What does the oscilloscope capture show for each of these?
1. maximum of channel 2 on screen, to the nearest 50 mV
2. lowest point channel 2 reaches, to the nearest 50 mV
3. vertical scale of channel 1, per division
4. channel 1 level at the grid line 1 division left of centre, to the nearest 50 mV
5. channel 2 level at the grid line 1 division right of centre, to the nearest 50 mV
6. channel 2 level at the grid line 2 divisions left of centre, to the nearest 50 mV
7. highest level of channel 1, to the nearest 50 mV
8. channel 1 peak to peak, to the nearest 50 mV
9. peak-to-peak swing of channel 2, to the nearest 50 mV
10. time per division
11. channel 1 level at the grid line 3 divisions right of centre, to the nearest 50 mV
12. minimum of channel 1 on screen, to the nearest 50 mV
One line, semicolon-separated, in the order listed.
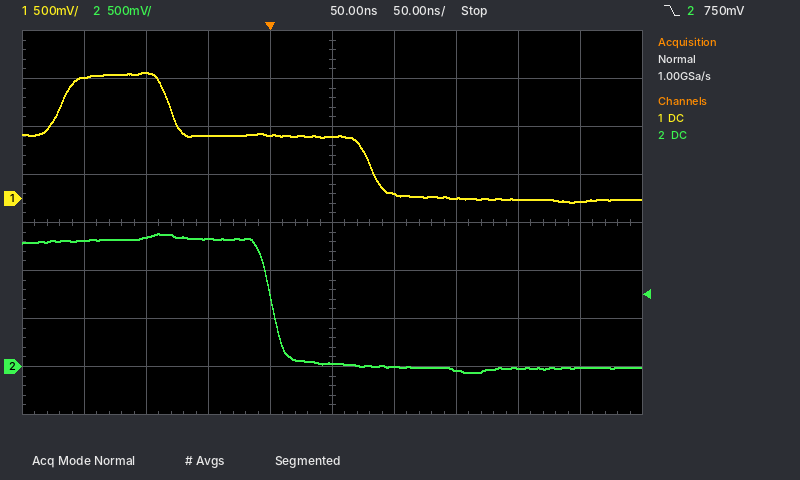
1.40 V; -50 mV; 500 mV; 650 mV; 0 mV; 1.35 V; 1.30 V; 1.35 V; 1.45 V; 50 ns; 0 mV; -50 mV
